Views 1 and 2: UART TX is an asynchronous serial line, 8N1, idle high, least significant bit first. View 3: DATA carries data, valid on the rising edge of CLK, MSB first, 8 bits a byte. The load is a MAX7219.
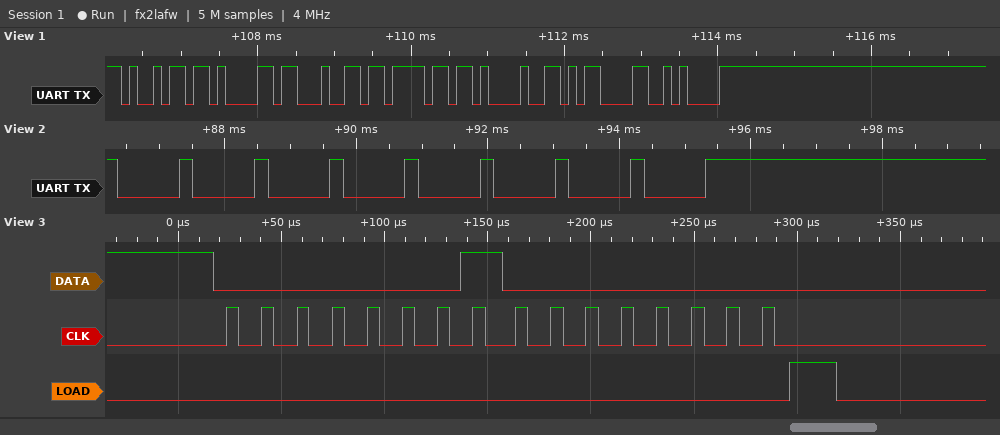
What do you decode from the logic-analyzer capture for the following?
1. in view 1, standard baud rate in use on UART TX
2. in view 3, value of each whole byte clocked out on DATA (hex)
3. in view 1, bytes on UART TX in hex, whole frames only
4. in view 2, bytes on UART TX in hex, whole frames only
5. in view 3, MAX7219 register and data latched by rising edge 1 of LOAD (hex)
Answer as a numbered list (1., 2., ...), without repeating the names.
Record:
1. 9600 baud
2. 01 00
3. 0x69 0x61 0x64 0x6F 0x21 0x0D 0x0A
4. 0x00 0x00 0x00 0x00 0x00 0x00 0x00 0x00
5. register 0x1, data 0x00
